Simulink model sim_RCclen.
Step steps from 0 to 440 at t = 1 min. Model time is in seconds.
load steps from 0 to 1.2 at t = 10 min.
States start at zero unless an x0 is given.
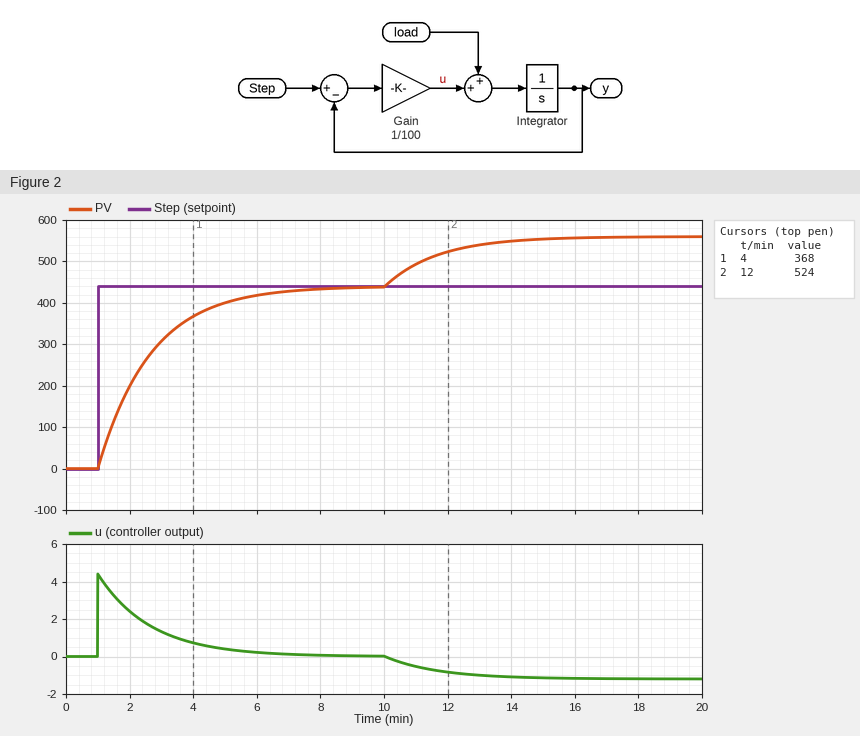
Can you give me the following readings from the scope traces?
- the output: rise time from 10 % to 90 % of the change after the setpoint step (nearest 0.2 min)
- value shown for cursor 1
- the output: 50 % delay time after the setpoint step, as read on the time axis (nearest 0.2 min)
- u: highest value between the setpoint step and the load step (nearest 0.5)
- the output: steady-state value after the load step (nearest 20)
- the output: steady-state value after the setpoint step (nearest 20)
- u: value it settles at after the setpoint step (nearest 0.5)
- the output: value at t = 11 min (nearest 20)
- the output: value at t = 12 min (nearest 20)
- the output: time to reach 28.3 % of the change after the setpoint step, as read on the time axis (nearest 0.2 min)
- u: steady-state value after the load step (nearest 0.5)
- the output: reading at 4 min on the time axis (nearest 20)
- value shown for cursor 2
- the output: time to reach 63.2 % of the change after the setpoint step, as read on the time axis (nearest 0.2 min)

3.6 min
368
2.2 min
4.5
560
440
0.0
500
520
1.6 min
-1.0
360
524
2.6 min
